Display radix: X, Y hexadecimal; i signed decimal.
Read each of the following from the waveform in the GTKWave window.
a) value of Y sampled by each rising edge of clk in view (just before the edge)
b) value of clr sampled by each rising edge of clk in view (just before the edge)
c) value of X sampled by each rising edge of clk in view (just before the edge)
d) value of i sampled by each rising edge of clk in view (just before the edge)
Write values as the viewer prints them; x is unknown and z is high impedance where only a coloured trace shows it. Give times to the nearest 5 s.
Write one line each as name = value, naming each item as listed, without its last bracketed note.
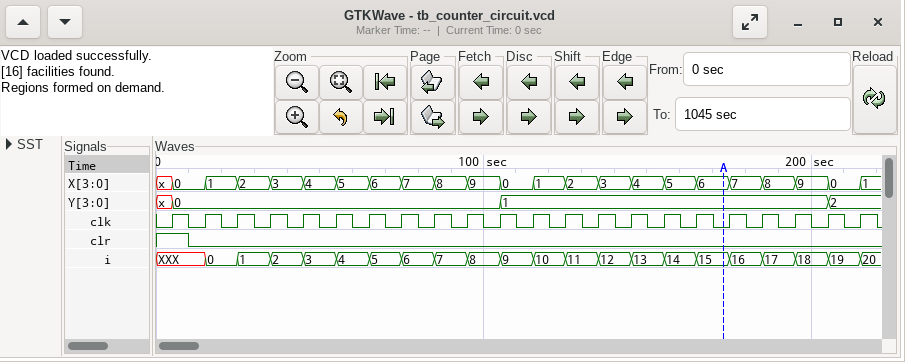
value of Y sampled by each rising edge of clk in view = x, 0, 0, 0, 0, 0, 0, 0, 0, 0, 0, 1, 1, 1, 1, 1, 1, 1, 1, 1, 1, 2
value of clr sampled by each rising edge of clk in view = 1 0 0 0 0 0 0 0 0 0 0 0 0 0 0 0 0 0 0 0 0 0
value of X sampled by each rising edge of clk in view = x, 0, 1, 2, 3, 4, 5, 6, 7, 8, 9, 0, 1, 2, 3, 4, 5, 6, 7, 8, 9, 0
value of i sampled by each rising edge of clk in view = XXX, XXX, 0, 1, 2, 3, 4, 5, 6, 7, 8, 9, 10, 11, 12, 13, 14, 15, 16, 17, 18, 19
